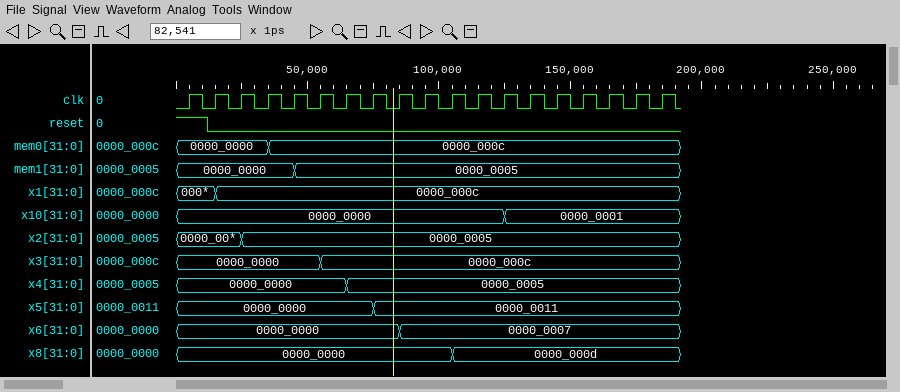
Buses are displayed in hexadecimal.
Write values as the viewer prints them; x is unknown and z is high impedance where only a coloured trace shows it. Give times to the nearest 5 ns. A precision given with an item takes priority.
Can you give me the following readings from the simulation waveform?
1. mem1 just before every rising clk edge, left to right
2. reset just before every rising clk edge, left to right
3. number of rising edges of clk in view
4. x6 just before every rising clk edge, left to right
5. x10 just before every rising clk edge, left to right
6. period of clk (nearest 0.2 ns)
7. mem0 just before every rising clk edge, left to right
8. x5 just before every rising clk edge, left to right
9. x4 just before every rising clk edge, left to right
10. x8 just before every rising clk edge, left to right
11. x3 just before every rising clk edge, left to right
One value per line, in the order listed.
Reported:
0000_0000, 0000_0000, 0000_0000, 0000_0000, 0000_0000, 0000_0005, 0000_0005, 0000_0005, 0000_0005, 0000_0005, 0000_0005, 0000_0005, 0000_0005, 0000_0005, 0000_0005, 0000_0005, 0000_0005, 0000_0005, 0000_0005
1 0 0 0 0 0 0 0 0 0 0 0 0 0 0 0 0 0 0
19
0000_0000, 0000_0000, 0000_0000, 0000_0000, 0000_0000, 0000_0000, 0000_0000, 0000_0000, 0000_0000, 0000_0007, 0000_0007, 0000_0007, 0000_0007, 0000_0007, 0000_0007, 0000_0007, 0000_0007, 0000_0007, 0000_0007
0000_0000, 0000_0000, 0000_0000, 0000_0000, 0000_0000, 0000_0000, 0000_0000, 0000_0000, 0000_0000, 0000_0000, 0000_0000, 0000_0000, 0000_0000, 0000_0001, 0000_0001, 0000_0001, 0000_0001, 0000_0001, 0000_0001
10 ns
0000_0000, 0000_0000, 0000_0000, 0000_0000, 0000_000c, 0000_000c, 0000_000c, 0000_000c, 0000_000c, 0000_000c, 0000_000c, 0000_000c, 0000_000c, 0000_000c, 0000_000c, 0000_000c, 0000_000c, 0000_000c, 0000_000c
0000_0000, 0000_0000, 0000_0000, 0000_0000, 0000_0000, 0000_0000, 0000_0000, 0000_0000, 0000_0011, 0000_0011, 0000_0011, 0000_0011, 0000_0011, 0000_0011, 0000_0011, 0000_0011, 0000_0011, 0000_0011, 0000_0011
0000_0000, 0000_0000, 0000_0000, 0000_0000, 0000_0000, 0000_0000, 0000_0000, 0000_0005, 0000_0005, 0000_0005, 0000_0005, 0000_0005, 0000_0005, 0000_0005, 0000_0005, 0000_0005, 0000_0005, 0000_0005, 0000_0005
0000_0000, 0000_0000, 0000_0000, 0000_0000, 0000_0000, 0000_0000, 0000_0000, 0000_0000, 0000_0000, 0000_0000, 0000_0000, 0000_000d, 0000_000d, 0000_000d, 0000_000d, 0000_000d, 0000_000d, 0000_000d, 0000_000d
0000_0000, 0000_0000, 0000_0000, 0000_0000, 0000_0000, 0000_0000, 0000_000c, 0000_000c, 0000_000c, 0000_000c, 0000_000c, 0000_000c, 0000_000c, 0000_000c, 0000_000c, 0000_000c, 0000_000c, 0000_000c, 0000_000c
